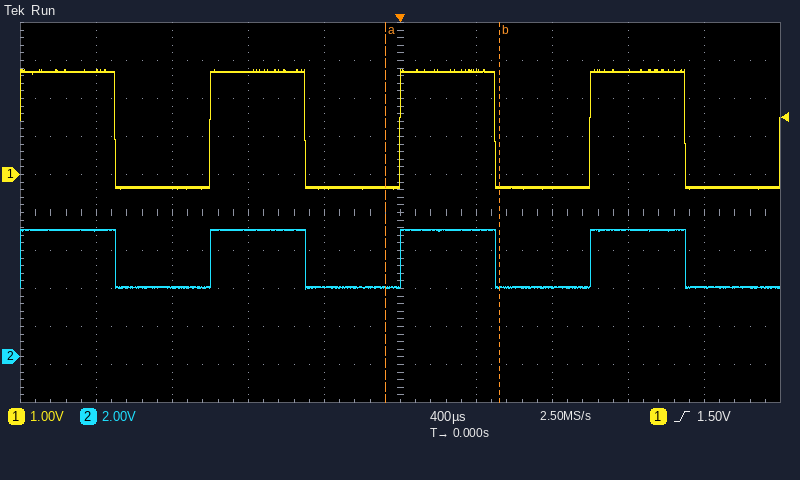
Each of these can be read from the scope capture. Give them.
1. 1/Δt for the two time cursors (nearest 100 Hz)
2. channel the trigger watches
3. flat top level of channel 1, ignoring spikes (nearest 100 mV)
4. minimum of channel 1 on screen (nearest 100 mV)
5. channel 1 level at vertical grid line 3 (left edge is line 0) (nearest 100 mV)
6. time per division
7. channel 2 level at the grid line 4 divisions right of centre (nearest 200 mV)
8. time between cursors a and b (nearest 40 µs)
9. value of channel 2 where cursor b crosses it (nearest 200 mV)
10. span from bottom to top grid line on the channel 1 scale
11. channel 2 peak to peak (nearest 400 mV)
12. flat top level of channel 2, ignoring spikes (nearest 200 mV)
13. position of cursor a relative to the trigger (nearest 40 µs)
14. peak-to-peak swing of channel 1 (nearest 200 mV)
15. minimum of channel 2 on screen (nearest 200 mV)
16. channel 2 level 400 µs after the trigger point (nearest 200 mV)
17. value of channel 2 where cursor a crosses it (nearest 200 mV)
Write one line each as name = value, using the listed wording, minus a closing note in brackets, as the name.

1/Δt for the two time cursors = 1.7 kHz
channel the trigger watches = channel 1
flat top level of channel 1, ignoring spikes = 2.7 V
minimum of channel 1 on screen = -400 mV
channel 1 level at vertical grid line 3 (left edge is line 0) = 2.7 V
time per division = 400 µs
channel 2 level at the grid line 4 divisions right of centre = 3.6 V
time between cursors a and b = 600 µs
value of channel 2 where cursor b crosses it = 3.6 V
span from bottom to top grid line on the channel 1 scale = 10 V
channel 2 peak to peak = 3.2 V
flat top level of channel 2, ignoring spikes = 6.6 V
position of cursor a relative to the trigger = -80 µs
peak-to-peak swing of channel 1 = 3.2 V
minimum of channel 2 on screen = 3.6 V
channel 2 level 400 µs after the trigger point = 6.6 V
value of channel 2 where cursor a crosses it = 3.6 V
